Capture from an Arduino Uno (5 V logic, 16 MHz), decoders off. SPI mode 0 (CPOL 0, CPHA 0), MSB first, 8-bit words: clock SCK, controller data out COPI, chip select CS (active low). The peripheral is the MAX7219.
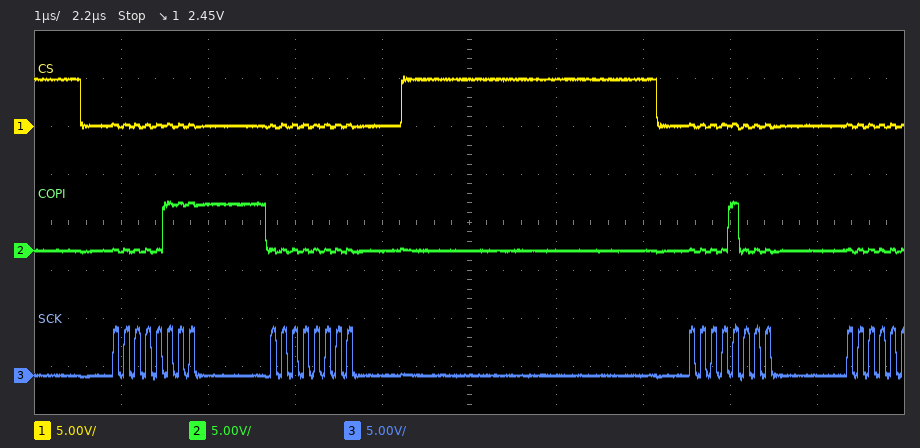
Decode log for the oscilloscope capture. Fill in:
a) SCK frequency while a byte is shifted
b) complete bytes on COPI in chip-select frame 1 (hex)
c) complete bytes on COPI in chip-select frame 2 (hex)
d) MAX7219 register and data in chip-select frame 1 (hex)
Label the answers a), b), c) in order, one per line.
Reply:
a) 8 MHz
b) 07 00
c) 08
d) register 0x7, data 0x00
